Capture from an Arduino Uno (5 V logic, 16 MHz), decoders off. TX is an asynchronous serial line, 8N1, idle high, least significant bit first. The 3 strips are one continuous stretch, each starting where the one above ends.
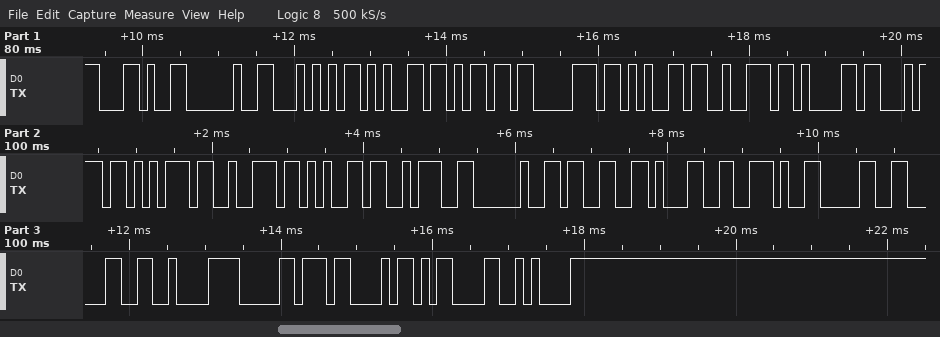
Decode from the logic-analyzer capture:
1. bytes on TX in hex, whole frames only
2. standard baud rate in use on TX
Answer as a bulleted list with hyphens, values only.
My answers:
- 2C 20 54 65 6D 70 65 72 61 74 75 72 65 3A 20 33 31 2E 30 30 C2 B0 43 0D 0A
- 9600 baud
